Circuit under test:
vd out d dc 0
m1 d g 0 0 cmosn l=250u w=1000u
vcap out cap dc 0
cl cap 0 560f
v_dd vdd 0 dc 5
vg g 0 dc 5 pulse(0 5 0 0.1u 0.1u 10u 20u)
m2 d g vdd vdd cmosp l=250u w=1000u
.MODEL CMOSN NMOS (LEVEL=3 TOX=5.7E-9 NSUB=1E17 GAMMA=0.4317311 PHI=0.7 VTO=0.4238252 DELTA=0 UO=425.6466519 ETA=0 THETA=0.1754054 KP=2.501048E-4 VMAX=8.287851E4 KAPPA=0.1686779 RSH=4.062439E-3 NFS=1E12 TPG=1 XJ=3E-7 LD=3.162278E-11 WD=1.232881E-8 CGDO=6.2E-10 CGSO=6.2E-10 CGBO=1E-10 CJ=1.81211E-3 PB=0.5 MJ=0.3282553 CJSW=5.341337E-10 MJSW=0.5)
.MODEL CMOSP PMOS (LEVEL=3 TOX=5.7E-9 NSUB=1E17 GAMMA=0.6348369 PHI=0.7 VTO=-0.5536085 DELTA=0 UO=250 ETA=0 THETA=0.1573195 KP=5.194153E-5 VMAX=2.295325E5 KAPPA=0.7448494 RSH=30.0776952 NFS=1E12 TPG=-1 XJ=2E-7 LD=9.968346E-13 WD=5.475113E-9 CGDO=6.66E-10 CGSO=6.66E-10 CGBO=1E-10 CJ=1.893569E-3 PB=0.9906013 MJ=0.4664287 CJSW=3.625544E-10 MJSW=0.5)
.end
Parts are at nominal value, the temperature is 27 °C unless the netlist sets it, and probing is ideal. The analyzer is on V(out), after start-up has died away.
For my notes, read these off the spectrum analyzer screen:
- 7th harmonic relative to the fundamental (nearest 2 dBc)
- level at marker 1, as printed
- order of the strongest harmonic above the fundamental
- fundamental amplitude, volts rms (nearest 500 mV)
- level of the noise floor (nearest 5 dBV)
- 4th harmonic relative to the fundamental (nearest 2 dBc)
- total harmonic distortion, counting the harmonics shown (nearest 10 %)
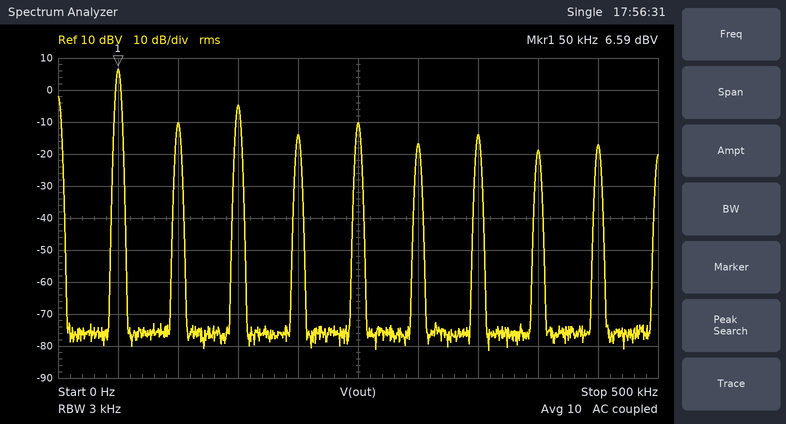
-20 dBc
6.59 dBV
3
2.0 V
-75 dBV
-20 dBc
40 %
